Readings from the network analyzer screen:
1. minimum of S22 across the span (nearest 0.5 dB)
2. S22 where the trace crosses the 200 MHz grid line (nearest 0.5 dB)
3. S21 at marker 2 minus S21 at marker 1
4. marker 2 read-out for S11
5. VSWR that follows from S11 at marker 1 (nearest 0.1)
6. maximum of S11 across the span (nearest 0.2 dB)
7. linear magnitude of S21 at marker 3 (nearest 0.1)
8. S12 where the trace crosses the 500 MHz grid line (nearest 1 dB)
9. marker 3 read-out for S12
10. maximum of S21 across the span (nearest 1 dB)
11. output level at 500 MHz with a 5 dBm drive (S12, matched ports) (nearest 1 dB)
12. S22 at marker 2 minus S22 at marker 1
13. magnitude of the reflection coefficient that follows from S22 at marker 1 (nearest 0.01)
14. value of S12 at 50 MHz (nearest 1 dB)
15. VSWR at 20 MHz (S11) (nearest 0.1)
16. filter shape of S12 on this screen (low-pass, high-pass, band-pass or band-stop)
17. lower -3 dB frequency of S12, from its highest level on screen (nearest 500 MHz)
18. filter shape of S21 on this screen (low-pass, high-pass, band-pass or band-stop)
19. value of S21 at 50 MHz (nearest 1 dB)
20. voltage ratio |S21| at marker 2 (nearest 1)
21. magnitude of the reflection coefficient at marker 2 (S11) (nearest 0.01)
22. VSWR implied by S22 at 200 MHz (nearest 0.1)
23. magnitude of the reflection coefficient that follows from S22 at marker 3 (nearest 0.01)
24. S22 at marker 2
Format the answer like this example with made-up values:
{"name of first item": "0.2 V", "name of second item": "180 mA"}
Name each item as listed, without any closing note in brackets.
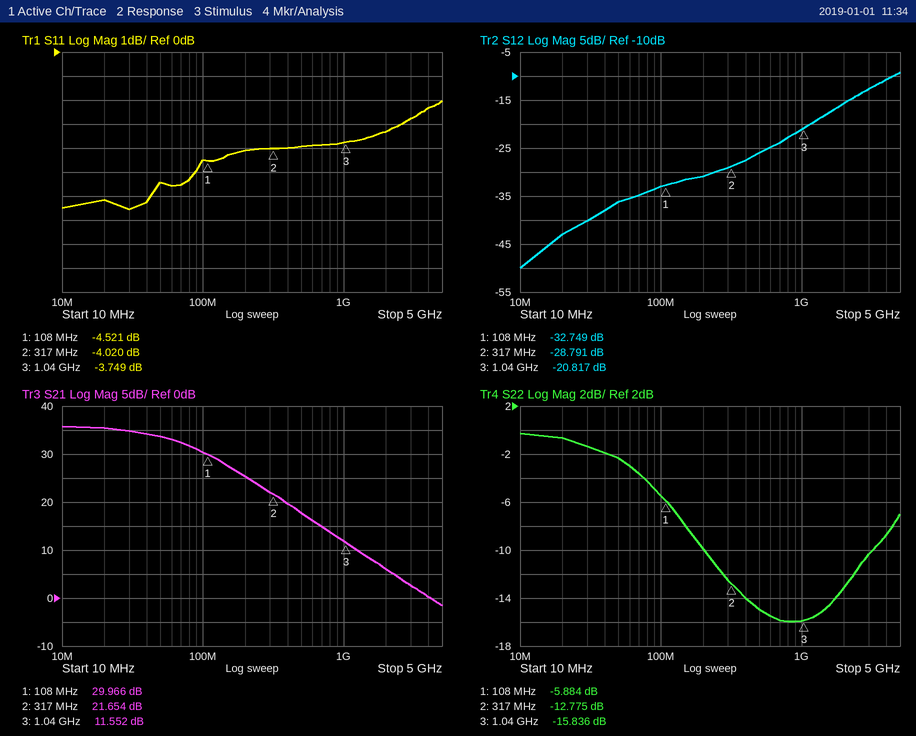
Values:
{"minimum of S22 across the span": "-16.0 dB", "S22 where the trace crosses the 200 MHz grid line": "-10.0 dB", "S21 at marker 2 minus S21 at marker 1": "-8.312 dB", "marker 2 read-out for S11": "-4.020 dB", "VSWR that follows from S11 at marker 1": "3.9", "maximum of S11 across the span": "-2.0 dB", "linear magnitude of S21 at marker 3": "3.8", "S12 where the trace crosses the 500 MHz grid line": "-26 dB", "marker 3 read-out for S12": "-20.817 dB", "maximum of S21 across the span": "36 dB", "output level at 500 MHz with a 5 dBm drive (S12, matched ports)": "-21 dBm", "S22 at marker 2 minus S22 at marker 1": "-6.891 dB", "magnitude of the reflection coefficient that follows from S22 at marker 1": "0.51", "value of S12 at 50 MHz": "-36 dB", "VSWR at 20 MHz (S11)": "2.9", "filter shape of S12 on this screen": "high-pass", "lower -3 dB frequency of S12, from its highest level on screen": "3.0 GHz", "filter shape of S21 on this screen": "low-pass", "value of S21 at 50 MHz": "34 dB", "voltage ratio |S21| at marker 2": "12", "magnitude of the reflection coefficient at marker 2 (S11)": "0.63", "VSWR implied by S22 at 200 MHz": "1.9", "magnitude of the reflection coefficient that follows from S22 at marker 3": "0.16", "S22 at marker 2": "-12.775 dB"}
